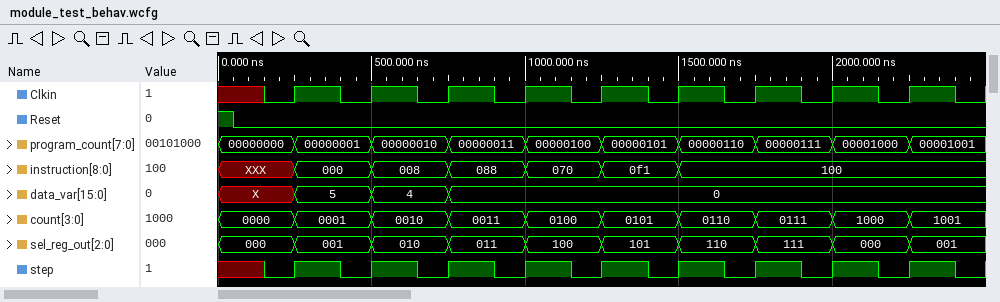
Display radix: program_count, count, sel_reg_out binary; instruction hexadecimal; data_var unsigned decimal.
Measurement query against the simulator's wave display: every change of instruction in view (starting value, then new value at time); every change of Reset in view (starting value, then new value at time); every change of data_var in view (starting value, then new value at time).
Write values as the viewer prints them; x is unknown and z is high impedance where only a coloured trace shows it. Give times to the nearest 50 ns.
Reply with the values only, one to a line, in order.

XXX, 000 at 250 ns, 008 at 500 ns, 088 at 750 ns, 070 at 1000 ns, 0f1 at 1250 ns, 100 at 1500 ns
1, 0 at 50 ns
X, 5 at 250 ns, 4 at 500 ns, 0 at 750 ns
